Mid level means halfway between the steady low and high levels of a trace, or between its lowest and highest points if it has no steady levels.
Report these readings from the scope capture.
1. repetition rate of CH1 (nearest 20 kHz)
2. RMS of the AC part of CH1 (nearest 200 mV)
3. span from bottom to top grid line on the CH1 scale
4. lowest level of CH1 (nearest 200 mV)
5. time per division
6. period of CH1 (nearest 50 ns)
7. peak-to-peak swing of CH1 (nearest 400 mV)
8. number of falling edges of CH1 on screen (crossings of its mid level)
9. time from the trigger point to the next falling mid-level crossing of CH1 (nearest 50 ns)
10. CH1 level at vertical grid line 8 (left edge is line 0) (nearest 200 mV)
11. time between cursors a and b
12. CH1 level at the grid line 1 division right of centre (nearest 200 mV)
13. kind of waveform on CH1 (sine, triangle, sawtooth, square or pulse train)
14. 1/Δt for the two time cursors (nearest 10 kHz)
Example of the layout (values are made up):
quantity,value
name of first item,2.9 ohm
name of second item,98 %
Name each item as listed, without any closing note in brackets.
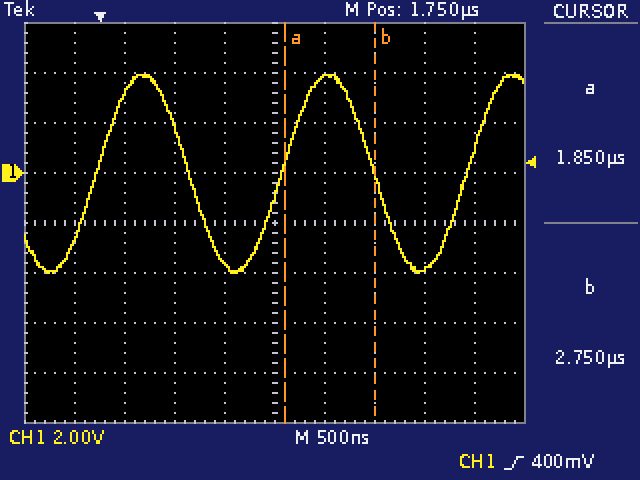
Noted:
quantity,value
repetition rate of CH1,540 kHz
RMS of the AC part of CH1,2.8 V
span from bottom to top grid line on the CH1 scale,16 V
lowest level of CH1,-4.0 V
time per division,500 ns
period of CH1,1.85 µs
peak-to-peak swing of CH1,8.0 V
number of falling edges of CH1 on screen,2
time from the trigger point to the next falling mid-level crossing of CH1,900 ns
CH1 level at vertical grid line 8 (left edge is line 0),-3.8 V
time between cursors a and b,900 ns
CH1 level at the grid line 1 division right of centre,3.8 V
kind of waveform on CH1,sine
1/Δt for the two time cursors,1.11 MHz
